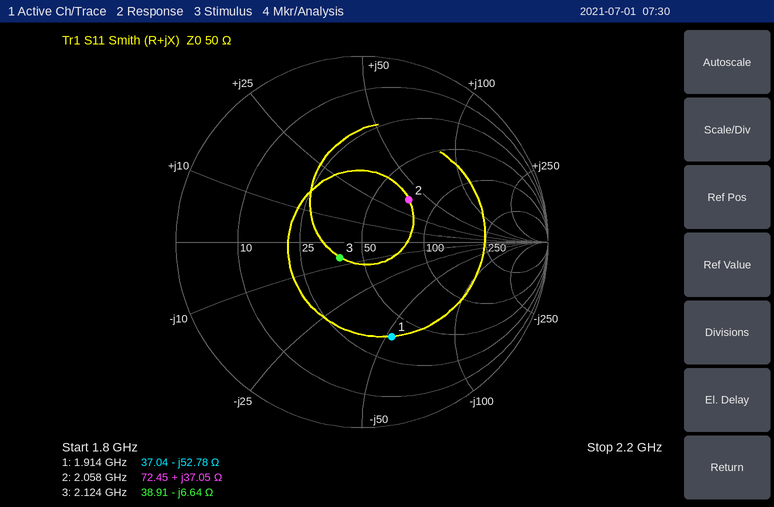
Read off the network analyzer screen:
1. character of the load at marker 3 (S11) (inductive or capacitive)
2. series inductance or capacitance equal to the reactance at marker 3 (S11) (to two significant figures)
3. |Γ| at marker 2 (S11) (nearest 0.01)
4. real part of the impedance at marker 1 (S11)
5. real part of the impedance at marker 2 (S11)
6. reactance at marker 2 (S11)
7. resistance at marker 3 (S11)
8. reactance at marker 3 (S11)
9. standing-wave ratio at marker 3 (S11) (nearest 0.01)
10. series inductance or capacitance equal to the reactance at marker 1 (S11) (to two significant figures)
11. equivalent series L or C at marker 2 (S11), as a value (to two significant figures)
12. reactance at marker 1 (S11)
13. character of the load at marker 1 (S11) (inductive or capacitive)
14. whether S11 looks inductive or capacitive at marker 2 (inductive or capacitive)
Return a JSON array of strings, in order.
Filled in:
["capacitive", "11 pF", "0.34", "37.04 Ω", "72.45 Ω", "+37.05 Ω", "38.91 Ω", "-6.64 Ω", "1.34", "1.6 pF", "2.9 nH", "-52.78 Ω", "capacitive", "inductive"]
